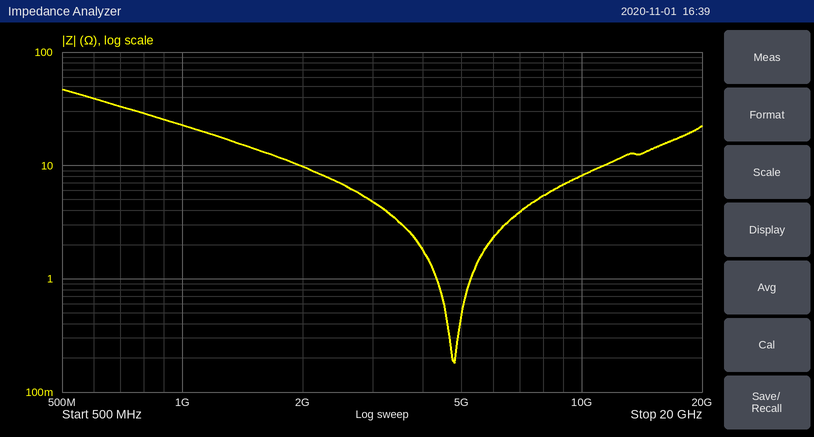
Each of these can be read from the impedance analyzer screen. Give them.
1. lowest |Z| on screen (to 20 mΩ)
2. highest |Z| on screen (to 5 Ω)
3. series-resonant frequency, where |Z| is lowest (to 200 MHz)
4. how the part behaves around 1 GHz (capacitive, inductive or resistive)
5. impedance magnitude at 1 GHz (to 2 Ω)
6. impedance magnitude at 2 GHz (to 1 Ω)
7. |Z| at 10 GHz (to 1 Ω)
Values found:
180 mΩ
45 Ω
4.8 GHz
capacitive
22 Ω
10 Ω
8 Ω
